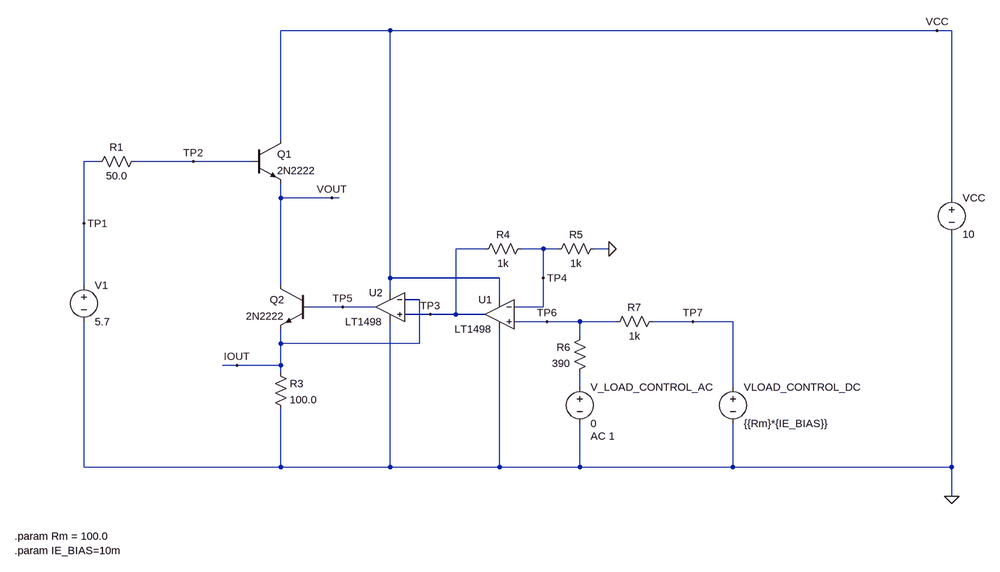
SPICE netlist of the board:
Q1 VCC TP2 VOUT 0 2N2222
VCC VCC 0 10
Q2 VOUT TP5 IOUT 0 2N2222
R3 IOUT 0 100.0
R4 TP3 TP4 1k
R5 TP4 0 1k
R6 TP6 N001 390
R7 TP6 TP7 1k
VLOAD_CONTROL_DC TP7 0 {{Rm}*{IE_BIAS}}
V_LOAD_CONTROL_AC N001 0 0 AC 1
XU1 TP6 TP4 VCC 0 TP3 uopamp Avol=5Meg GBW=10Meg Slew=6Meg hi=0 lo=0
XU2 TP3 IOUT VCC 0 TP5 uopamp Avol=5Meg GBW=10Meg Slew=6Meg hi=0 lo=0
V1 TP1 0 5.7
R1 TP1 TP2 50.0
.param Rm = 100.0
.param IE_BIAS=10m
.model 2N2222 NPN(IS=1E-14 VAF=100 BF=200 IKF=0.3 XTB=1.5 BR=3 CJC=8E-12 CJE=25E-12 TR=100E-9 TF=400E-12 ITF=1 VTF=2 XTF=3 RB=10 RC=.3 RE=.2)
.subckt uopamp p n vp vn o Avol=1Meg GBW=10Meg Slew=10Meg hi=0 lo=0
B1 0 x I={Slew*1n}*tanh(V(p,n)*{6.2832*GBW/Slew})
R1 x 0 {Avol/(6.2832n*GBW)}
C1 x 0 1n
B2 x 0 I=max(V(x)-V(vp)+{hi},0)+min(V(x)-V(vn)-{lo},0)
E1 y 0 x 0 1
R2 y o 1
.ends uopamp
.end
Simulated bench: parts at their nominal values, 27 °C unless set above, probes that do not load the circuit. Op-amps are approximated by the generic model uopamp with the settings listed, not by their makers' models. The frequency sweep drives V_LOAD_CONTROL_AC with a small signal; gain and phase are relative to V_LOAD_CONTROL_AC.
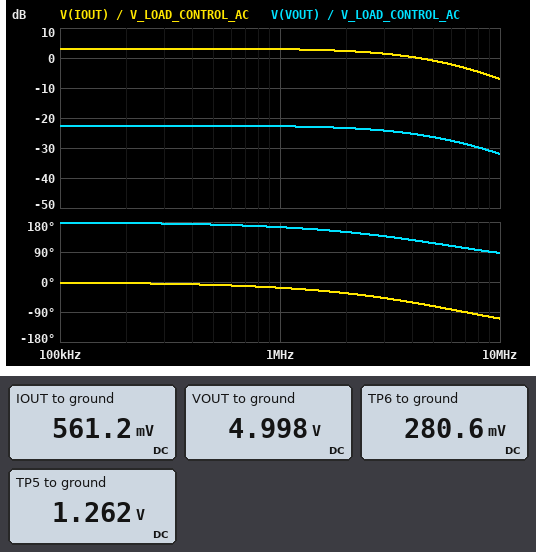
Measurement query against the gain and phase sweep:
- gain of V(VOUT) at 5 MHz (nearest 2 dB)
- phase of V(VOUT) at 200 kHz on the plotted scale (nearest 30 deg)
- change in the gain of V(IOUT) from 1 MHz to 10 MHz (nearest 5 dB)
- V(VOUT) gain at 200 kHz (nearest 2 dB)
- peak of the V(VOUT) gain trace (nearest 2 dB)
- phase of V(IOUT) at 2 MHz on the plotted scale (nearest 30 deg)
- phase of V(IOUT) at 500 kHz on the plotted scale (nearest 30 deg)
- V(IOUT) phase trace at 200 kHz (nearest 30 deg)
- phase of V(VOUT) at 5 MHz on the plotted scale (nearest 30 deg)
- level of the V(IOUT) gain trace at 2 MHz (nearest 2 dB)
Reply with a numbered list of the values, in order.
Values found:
1. -26 dB
2. 180 deg
3. -10 dB
4. -22 dB
5. -22 dB
6. -30 deg
7. 0 deg
8. 0 deg
9. 120 deg
10. 2 dB
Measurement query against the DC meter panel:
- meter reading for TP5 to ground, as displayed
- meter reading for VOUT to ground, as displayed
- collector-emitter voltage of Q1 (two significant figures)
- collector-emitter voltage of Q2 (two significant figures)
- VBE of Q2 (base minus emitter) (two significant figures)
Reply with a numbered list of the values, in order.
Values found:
1. 1.262 V
2. 4.998 V
3. 5.0 V
4. 4.4 V
5. 700 mV
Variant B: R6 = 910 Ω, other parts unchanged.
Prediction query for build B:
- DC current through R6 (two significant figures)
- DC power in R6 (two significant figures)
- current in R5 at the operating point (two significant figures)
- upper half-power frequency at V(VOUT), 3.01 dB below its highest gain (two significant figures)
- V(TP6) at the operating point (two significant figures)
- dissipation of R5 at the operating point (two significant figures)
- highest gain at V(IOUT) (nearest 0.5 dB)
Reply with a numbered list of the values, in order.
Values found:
1. 520 µA
2. 250 µW
3. 480 µA
4. 4.4 MHz
5. 480 mV
6. 230 µW
7. 0.5 dB
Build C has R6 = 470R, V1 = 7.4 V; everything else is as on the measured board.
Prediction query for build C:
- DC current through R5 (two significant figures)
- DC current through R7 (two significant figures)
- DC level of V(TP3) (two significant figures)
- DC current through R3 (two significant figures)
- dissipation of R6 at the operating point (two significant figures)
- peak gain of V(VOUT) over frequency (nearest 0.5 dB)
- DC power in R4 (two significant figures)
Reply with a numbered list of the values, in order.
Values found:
1. 320 µA
2. 680 µA
3. 640 mV
4. 6.4 mA
5. 220 µW
6. -24.0 dB
7. 100 µW
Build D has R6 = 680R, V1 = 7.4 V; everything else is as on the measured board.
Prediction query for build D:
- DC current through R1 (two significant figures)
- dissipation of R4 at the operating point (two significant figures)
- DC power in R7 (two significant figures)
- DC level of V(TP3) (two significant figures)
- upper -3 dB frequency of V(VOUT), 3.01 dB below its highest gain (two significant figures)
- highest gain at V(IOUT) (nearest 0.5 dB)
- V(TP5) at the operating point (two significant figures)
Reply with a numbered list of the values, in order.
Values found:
1. 40 µA
2. 160 µW
3. 350 µW
4. 810 mV
5. 4.4 MHz
6. 1.5 dB
7. 1.5 V
